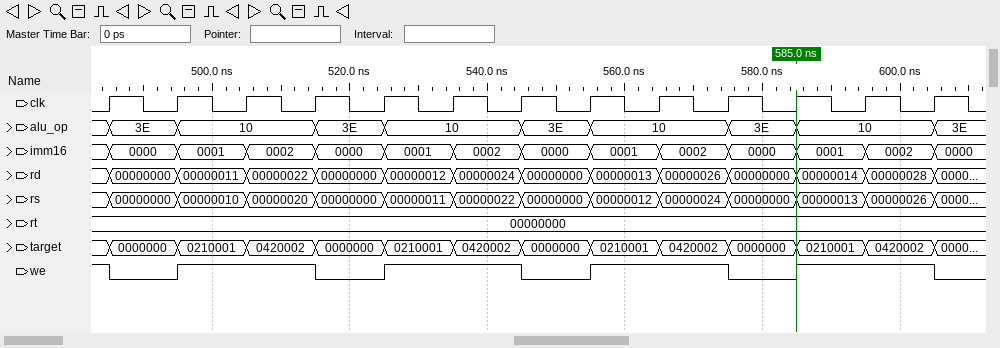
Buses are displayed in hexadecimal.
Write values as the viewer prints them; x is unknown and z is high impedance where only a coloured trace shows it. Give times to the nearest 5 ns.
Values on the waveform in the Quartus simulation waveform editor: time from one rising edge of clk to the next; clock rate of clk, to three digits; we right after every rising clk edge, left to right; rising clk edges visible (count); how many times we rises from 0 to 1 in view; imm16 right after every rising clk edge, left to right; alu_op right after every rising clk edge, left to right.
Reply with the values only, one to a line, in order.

10 ns
100 MHz
0 1 1 0 1 1 0 1 1 0 1 1 0
13
4
0000, 0001, 0002, 0000, 0001, 0002, 0000, 0001, 0002, 0000, 0001, 0002, 0000
3E, 10, 10, 3E, 10, 10, 3E, 10, 10, 3E, 10, 10, 3E
